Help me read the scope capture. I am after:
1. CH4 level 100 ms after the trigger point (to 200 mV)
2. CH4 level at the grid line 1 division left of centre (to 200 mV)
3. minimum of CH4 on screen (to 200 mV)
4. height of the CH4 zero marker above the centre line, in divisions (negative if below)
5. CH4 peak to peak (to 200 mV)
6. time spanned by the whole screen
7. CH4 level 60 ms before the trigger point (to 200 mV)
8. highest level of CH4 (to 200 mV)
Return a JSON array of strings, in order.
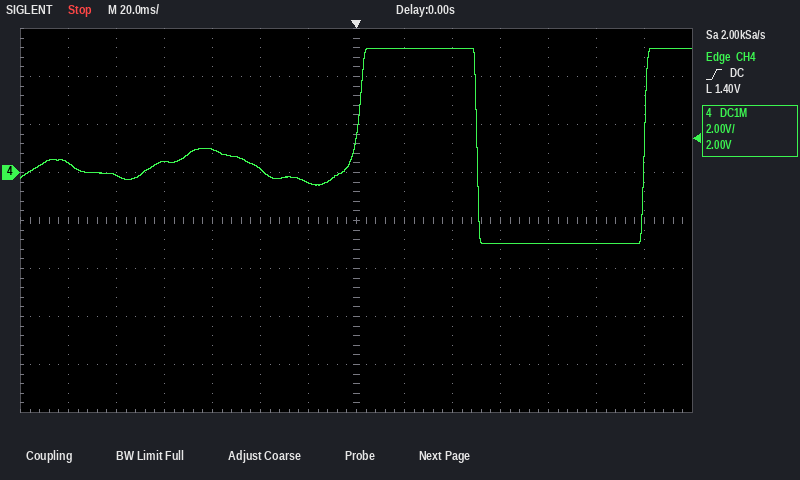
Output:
["-3.0 V", "-400 mV", "-3.0 V", "+1.0 div", "8.2 V", "280 ms", "1.0 V", "5.2 V"]
